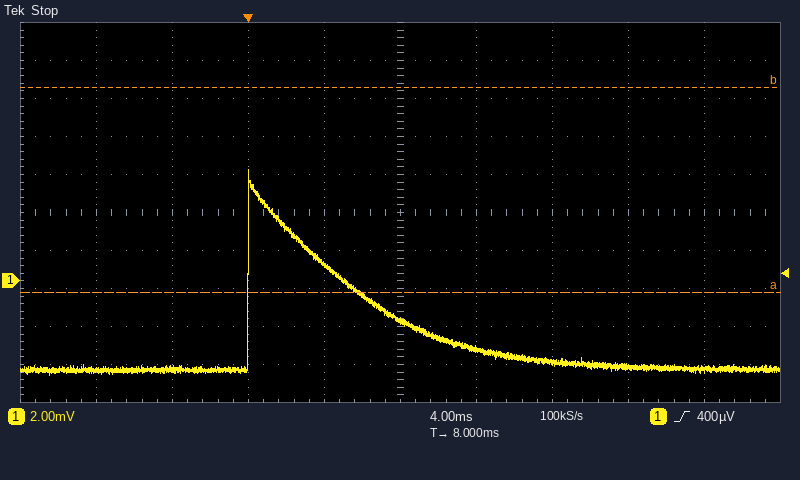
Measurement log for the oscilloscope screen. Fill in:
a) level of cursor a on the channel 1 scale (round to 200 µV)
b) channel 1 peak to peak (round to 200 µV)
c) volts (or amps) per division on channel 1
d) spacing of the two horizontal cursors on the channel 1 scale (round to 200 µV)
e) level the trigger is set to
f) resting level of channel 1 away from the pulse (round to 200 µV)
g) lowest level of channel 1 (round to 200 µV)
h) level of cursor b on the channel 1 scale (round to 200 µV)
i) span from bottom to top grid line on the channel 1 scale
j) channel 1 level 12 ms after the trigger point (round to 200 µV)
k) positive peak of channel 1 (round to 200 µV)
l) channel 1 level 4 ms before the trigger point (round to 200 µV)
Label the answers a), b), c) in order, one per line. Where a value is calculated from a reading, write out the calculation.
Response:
a) -600 µV
b) 5.8 mV − (-5.0 mV) = 10.8 mV
c) 2 mV
d) 10.8 mV
e) 400 µV
f) -4.6 mV
g) -5.0 mV
h) 10.2 mV
i) 20 mV
j) -3.6 mV
k) 5.8 mV
l) -4.6 mV
